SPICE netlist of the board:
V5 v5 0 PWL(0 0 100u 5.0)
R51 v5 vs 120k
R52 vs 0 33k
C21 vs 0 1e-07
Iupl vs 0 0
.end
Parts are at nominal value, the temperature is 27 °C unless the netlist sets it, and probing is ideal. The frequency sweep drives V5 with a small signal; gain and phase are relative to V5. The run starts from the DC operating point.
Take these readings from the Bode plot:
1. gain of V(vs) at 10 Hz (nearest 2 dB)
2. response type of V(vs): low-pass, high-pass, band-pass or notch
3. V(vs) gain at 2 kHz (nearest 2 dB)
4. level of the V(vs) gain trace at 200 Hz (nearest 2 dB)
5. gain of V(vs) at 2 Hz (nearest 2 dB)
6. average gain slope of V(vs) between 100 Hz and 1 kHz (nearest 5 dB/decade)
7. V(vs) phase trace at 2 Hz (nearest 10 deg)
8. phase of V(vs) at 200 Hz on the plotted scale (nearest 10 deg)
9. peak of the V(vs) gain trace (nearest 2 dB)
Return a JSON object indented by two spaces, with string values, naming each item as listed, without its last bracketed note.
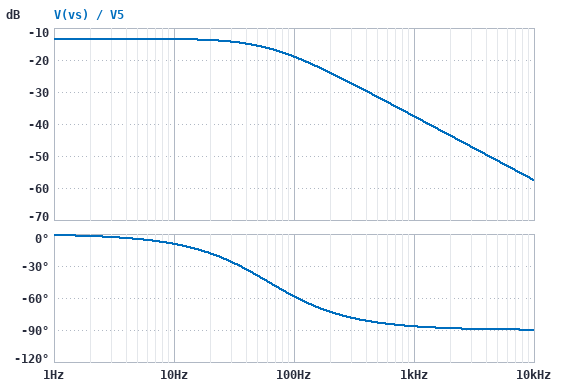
{
  "gain of V(vs) at 10 Hz": "-14 dB",
  "response type of V(vs): low-pass, high-pass, band-pass or notch": "low-pass",
  "V(vs) gain at 2 kHz": "-44 dB",
  "level of the V(vs) gain trace at 200 Hz": "-24 dB",
  "gain of V(vs) at 2 Hz": "-14 dB",
  "average gain slope of V(vs) between 100 Hz and 1 kHz": "-20 dB/decade",
  "V(vs) phase trace at 2 Hz": "0 deg",
  "phase of V(vs) at 200 Hz on the plotted scale": "-70 deg",
  "peak of the V(vs) gain trace": "-14 dB"
}
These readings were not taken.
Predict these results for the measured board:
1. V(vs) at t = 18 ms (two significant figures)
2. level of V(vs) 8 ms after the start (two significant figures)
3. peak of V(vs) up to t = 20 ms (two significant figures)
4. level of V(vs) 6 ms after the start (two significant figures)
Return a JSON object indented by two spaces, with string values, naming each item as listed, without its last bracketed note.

{
  "V(vs) at t = 18 ms": "1.1 V",
  "level of V(vs) 8 ms after the start": "1.0 V",
  "peak of V(vs) up to t = 20 ms": "1.1 V",
  "level of V(vs) 6 ms after the start": "970 mV"
}
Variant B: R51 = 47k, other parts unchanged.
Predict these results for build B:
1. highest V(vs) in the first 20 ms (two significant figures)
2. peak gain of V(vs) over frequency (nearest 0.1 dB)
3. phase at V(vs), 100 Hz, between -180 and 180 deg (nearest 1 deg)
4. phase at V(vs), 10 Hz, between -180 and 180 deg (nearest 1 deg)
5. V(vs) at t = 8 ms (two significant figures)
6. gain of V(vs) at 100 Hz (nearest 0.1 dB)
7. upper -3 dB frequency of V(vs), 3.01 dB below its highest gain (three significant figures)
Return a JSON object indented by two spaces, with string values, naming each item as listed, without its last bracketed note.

{
  "highest V(vs) in the first 20 ms": "2.1 V",
  "peak gain of V(vs) over frequency": "-7.7 dB",
  "phase at V(vs), 100 Hz, between -180 and 180 deg": "-51 deg",
  "phase at V(vs), 10 Hz, between -180 and 180 deg": "-7 deg",
  "V(vs) at t = 8 ms": "2.0 V",
  "gain of V(vs) at 100 Hz": "-11.6 dB",
  "upper -3 dB frequency of V(vs), 3.01 dB below its highest gain": "82.1 Hz"
}
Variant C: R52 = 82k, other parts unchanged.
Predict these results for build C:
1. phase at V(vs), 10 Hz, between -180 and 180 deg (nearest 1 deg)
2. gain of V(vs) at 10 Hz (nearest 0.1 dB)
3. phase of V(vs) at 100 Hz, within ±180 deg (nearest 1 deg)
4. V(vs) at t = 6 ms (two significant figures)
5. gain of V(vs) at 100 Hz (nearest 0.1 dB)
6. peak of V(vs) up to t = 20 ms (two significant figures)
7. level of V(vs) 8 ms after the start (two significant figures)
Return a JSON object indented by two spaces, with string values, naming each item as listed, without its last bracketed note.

{
  "phase at V(vs), 10 Hz, between -180 and 180 deg": "-17 deg",
  "gain of V(vs) at 10 Hz": "-8.2 dB",
  "phase of V(vs) at 100 Hz, within ±180 deg": "-72 deg",
  "V(vs) at t = 6 ms": "1.4 V",
  "gain of V(vs) at 100 Hz": "-18.0 dB",
  "peak of V(vs) up to t = 20 ms": "2.0 V",
  "level of V(vs) 8 ms after the start": "1.6 V"
}
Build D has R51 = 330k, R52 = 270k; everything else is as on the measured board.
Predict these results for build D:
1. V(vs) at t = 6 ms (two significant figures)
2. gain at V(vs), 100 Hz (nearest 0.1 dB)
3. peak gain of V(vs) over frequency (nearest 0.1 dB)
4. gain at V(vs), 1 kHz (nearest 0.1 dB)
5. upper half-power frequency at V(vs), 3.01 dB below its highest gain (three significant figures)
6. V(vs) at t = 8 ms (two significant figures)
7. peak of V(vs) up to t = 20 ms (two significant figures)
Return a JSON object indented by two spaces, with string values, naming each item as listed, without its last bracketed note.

{
  "V(vs) at t = 6 ms": "740 mV",
  "gain at V(vs), 100 Hz": "-26.4 dB",
  "peak gain of V(vs) over frequency": "-6.9 dB",
  "gain at V(vs), 1 kHz": "-46.3 dB",
  "upper half-power frequency at V(vs), 3.01 dB below its highest gain": "10.7 Hz",
  "V(vs) at t = 8 ms": "930 mV",
  "peak of V(vs) up to t = 20 ms": "1.7 V"
}
